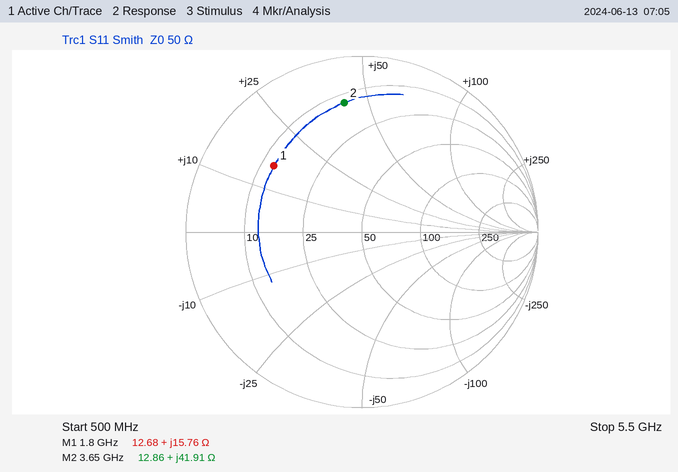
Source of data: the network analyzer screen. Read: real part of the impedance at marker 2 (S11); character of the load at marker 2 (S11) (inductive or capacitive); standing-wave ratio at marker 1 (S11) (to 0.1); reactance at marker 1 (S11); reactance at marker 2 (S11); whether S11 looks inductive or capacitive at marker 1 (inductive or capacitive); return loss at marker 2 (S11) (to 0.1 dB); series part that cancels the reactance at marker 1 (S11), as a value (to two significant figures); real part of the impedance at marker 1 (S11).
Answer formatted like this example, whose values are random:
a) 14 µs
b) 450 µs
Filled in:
a) 12.86 Ω
b) inductive
c) 4.4
d) +15.76 Ω
e) +41.91 Ω
f) inductive
g) 2.6 dB
h) 5.6 pF
i) 12.68 Ω
